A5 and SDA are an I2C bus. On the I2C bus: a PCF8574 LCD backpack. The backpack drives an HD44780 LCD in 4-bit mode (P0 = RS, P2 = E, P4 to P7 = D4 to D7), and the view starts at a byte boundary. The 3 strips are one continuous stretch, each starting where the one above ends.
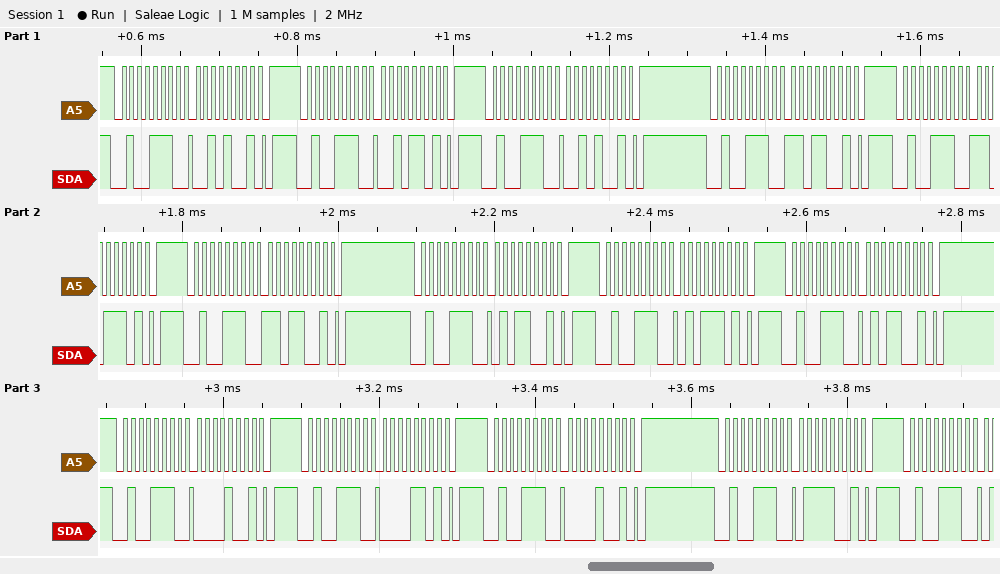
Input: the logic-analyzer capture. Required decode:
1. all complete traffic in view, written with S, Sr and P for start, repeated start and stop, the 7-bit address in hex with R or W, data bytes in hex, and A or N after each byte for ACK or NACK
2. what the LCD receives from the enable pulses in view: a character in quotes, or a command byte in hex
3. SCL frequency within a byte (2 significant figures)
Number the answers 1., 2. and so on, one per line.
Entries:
1. S 27W A 29 A P S 27W A 2D A P S 27W A 29 A P S 27W A D9 A P S 27W A DD A P S 27W A D9 A P S 27W A 59 A P S 27W A 5D A P S 27W A 59 A P S 27W A 09 A P S 27W A 0D A P S 27W A 09 A P S 27W A 79 A P S 27W A
2. '-' 'P'
3. 100 kHz
